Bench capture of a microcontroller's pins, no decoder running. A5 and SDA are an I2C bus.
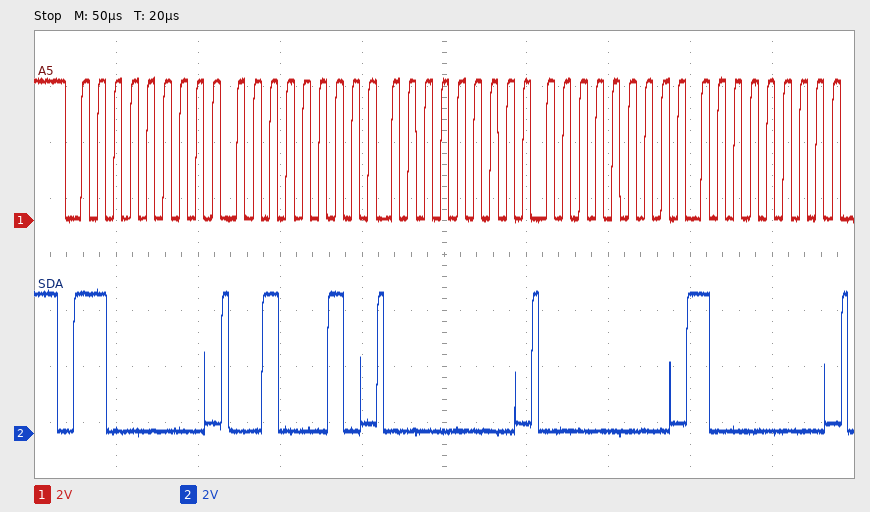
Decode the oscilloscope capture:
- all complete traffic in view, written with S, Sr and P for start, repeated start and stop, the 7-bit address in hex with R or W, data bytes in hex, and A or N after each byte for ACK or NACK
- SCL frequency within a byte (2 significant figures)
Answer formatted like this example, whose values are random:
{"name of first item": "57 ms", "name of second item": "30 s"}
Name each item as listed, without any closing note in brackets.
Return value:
{"all complete traffic in view, written with S, Sr and P for start, repeated start and stop, the 7-bit address in hex with R or W, data bytes in hex, and A or N after each byte for ACK or NACK": "S 60W A 22 A 00 A 00 A 80 A", "SCL frequency within a byte": "100 kHz"}
